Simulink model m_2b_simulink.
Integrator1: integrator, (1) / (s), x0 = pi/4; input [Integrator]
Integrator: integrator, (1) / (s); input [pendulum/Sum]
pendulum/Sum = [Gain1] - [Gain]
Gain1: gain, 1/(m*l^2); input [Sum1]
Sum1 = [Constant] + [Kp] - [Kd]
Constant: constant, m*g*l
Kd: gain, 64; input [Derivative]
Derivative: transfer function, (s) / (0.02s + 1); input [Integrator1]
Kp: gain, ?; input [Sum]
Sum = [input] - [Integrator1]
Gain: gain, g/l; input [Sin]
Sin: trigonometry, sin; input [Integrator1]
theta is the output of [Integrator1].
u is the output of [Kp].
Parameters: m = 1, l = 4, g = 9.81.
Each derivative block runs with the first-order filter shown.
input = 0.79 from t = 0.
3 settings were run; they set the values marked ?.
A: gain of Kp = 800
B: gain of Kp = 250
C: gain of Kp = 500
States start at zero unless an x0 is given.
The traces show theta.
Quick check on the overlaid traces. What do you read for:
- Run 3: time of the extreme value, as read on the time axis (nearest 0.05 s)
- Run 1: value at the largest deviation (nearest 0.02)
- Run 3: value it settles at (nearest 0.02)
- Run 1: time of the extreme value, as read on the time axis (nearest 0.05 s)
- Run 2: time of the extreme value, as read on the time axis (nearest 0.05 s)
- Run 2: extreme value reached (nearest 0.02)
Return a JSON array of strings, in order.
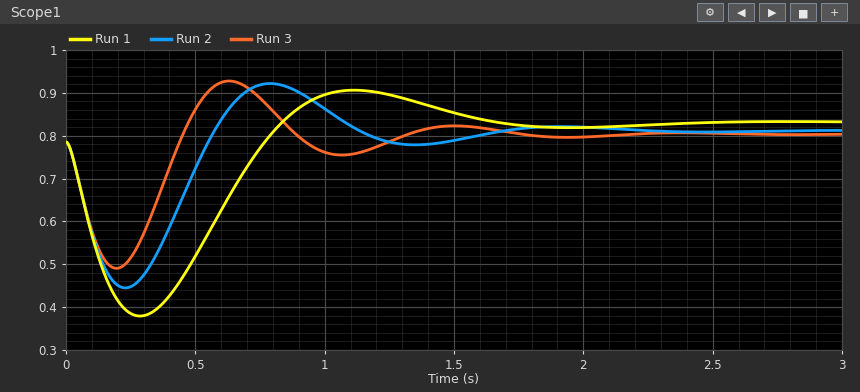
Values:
["0.20 s", "0.38", "0.80", "0.30 s", "0.25 s", "0.44"]
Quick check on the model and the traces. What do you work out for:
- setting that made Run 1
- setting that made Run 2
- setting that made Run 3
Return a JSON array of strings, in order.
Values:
["B", "C", "A"]
